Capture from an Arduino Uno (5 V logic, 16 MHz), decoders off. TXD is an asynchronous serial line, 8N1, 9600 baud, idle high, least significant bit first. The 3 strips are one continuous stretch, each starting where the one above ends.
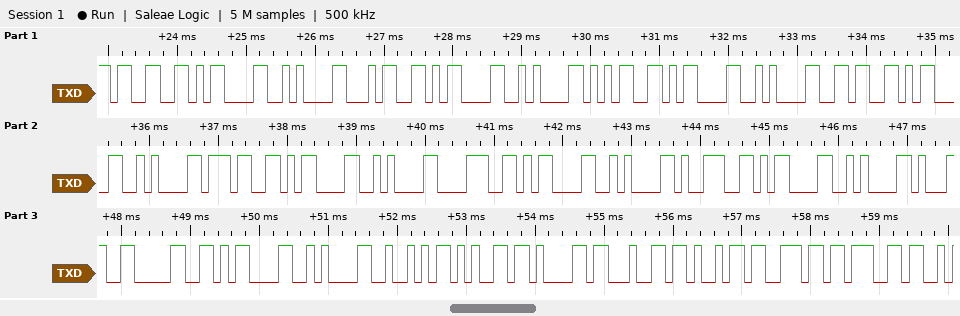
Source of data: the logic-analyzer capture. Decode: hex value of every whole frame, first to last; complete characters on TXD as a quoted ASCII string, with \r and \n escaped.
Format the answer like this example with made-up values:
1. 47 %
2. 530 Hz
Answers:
1. 33 0D 0A 34 0D 0A 35 0D 0A 36 0D 0A 37 0D 0A 38 0D 0A 39 0D 0A 31 30 0D 0A 52 65 61 64 69 6E 67
2. "3\r\n4\r\n5\r\n6\r\n7\r\n8\r\n9\r\n10\r\nReading"
